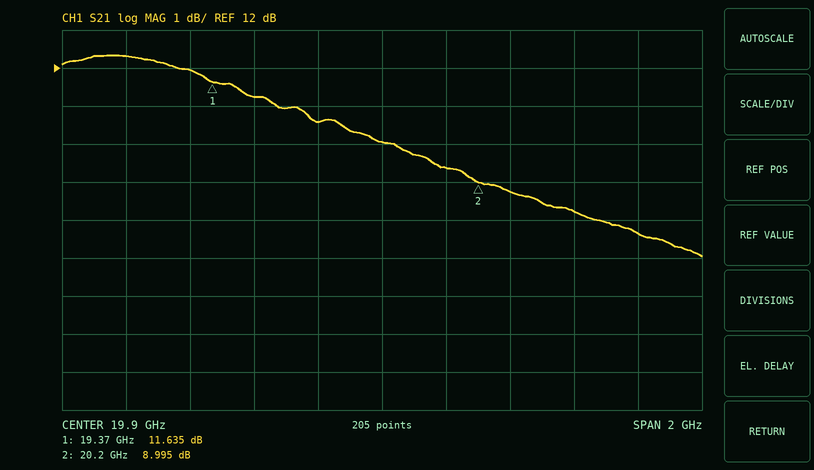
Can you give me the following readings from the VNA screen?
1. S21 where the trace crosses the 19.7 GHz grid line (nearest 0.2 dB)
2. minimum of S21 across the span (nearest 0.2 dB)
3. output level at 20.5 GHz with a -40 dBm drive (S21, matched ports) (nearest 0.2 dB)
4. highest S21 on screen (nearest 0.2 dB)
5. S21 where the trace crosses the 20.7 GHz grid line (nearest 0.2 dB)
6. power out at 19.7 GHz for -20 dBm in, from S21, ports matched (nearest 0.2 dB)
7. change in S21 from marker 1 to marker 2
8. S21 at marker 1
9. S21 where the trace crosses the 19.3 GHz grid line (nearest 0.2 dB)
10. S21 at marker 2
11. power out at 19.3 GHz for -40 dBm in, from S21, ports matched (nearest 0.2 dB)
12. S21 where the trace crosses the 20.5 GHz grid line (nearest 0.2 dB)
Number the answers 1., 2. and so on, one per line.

1. 10.6 dB
2. 7.0 dB
3. -31.8 dBm
4. 12.4 dB
5. 7.6 dB
6. -9.4 dBm
7. -2.640 dB
8. 11.635 dB
9. 12.0 dB
10. 8.995 dB
11. -28.0 dBm
12. 8.2 dB
